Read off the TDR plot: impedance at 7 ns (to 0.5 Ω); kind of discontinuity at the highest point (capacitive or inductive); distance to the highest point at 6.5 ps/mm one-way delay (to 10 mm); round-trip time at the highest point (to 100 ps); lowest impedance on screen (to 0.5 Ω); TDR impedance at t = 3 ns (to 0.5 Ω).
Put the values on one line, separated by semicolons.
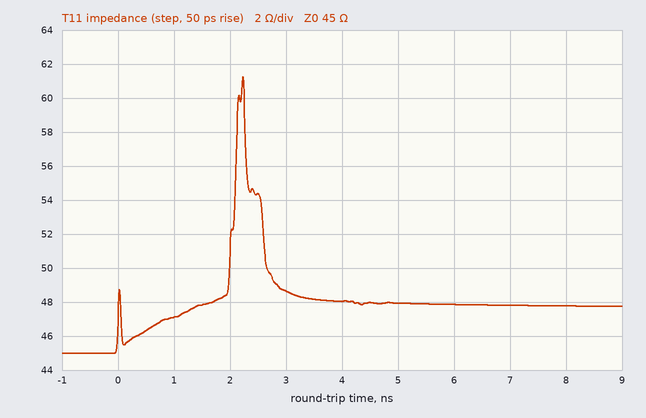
48.0 Ω; inductive; 170 mm; 2.2 ns; 45.0 Ω; 48.5 Ω
